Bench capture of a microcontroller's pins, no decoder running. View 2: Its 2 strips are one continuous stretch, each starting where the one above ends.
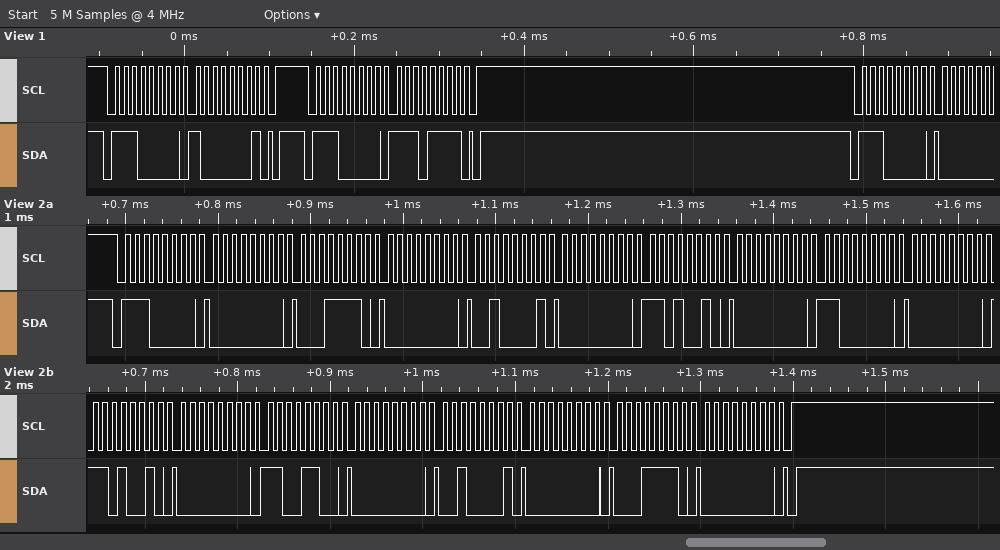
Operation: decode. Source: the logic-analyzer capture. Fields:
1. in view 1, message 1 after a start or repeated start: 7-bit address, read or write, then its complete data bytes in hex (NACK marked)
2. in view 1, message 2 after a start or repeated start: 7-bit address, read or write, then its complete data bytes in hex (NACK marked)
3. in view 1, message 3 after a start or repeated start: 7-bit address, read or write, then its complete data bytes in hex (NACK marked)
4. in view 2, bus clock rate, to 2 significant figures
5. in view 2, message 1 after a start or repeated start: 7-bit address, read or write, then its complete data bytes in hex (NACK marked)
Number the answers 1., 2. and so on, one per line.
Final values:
1. 0x70 write: 81
2. 0x70 write: EF
3. 0x70 write
4. 100 kHz
5. 0x70 write: 00 1E 00 21 00 D2 00 C0 00 D2 00 CC 00 21 00 1E 00
